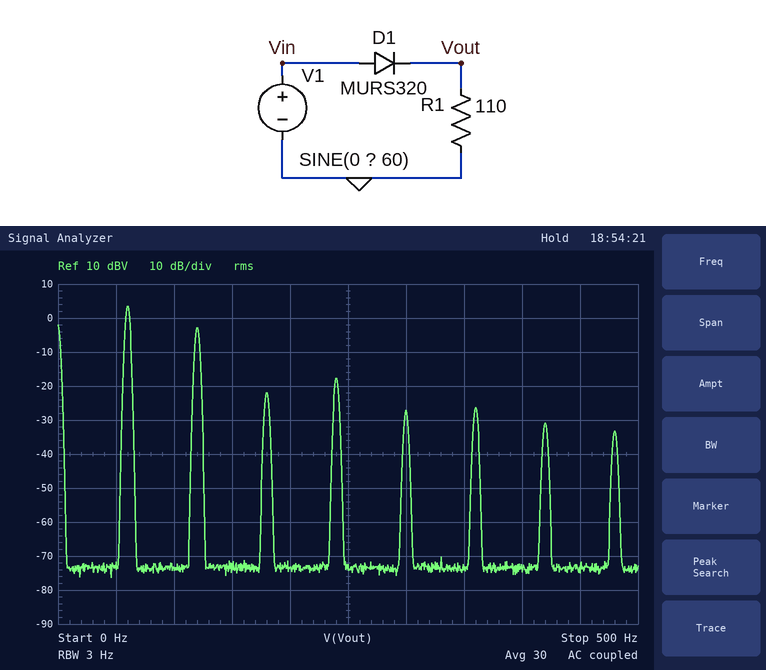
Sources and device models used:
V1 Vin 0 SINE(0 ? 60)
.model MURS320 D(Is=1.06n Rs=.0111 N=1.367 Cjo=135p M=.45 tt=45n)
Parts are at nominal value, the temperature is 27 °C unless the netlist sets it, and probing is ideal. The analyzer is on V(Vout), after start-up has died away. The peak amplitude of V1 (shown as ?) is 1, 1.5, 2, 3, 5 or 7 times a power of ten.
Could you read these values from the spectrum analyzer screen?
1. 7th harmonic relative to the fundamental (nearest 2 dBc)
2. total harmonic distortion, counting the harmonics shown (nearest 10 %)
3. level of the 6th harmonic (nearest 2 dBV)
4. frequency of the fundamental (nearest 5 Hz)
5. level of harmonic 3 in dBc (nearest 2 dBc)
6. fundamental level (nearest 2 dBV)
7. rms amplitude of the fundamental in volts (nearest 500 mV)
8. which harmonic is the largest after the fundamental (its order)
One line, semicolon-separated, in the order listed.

-34 dBc; 50 %; -26 dBV; 60 Hz; -26 dBc; 4 dBV; 1.5 V; 2
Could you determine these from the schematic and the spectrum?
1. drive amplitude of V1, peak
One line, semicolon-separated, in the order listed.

5 V
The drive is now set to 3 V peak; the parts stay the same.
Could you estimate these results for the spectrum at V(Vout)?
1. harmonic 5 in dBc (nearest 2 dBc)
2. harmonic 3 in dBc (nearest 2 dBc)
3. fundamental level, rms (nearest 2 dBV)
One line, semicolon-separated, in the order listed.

-26 dBc; -20 dBc; -2 dBV
